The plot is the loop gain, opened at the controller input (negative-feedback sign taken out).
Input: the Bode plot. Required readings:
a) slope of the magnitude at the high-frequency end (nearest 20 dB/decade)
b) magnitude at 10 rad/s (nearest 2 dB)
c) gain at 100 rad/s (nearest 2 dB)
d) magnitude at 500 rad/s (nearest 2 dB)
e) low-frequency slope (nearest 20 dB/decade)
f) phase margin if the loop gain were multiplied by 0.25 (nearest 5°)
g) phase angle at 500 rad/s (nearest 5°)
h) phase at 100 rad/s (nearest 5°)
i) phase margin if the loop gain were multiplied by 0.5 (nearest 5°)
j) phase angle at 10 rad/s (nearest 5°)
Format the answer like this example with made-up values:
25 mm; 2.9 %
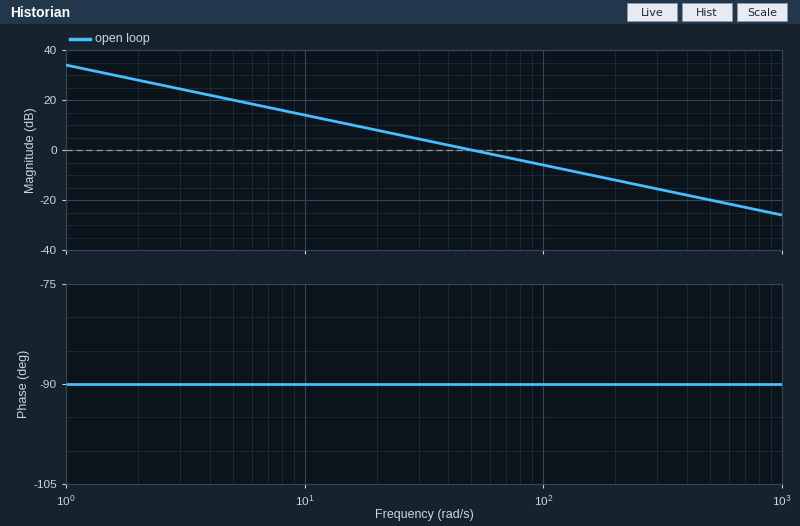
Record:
-20 dB/decade; 14 dB; -6 dB; -20 dB; -20 dB/decade; 90°; -90°; -90°; 90°; -90°
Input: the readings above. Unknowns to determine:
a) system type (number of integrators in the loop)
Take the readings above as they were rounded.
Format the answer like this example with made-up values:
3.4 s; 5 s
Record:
1
